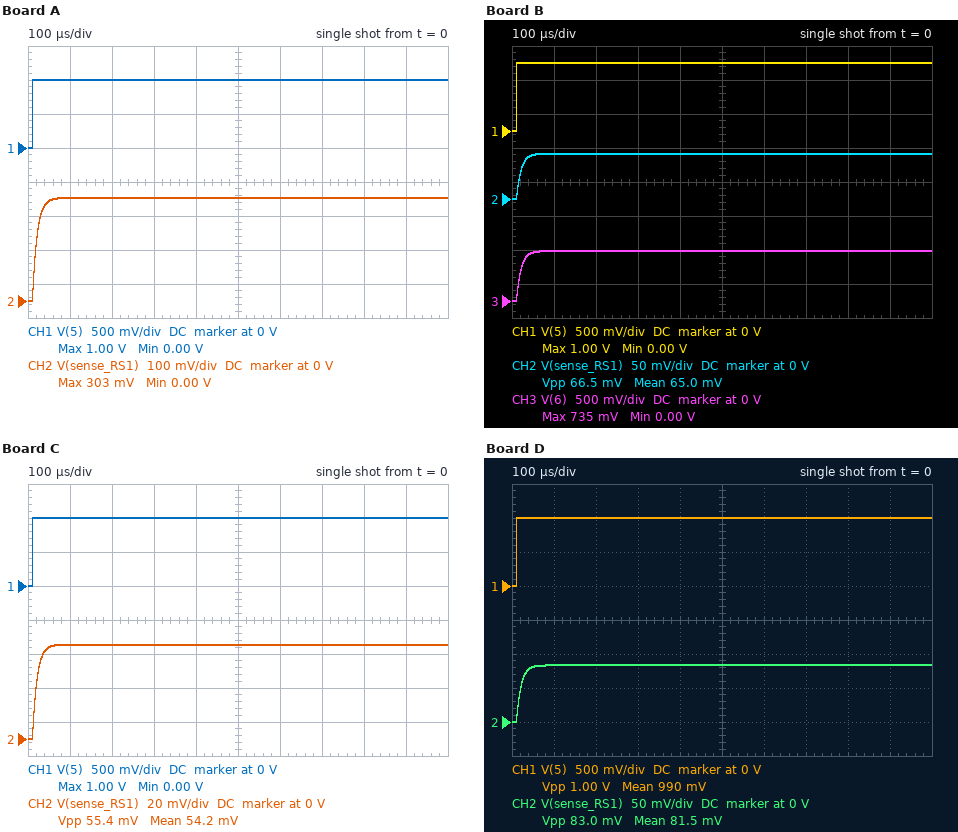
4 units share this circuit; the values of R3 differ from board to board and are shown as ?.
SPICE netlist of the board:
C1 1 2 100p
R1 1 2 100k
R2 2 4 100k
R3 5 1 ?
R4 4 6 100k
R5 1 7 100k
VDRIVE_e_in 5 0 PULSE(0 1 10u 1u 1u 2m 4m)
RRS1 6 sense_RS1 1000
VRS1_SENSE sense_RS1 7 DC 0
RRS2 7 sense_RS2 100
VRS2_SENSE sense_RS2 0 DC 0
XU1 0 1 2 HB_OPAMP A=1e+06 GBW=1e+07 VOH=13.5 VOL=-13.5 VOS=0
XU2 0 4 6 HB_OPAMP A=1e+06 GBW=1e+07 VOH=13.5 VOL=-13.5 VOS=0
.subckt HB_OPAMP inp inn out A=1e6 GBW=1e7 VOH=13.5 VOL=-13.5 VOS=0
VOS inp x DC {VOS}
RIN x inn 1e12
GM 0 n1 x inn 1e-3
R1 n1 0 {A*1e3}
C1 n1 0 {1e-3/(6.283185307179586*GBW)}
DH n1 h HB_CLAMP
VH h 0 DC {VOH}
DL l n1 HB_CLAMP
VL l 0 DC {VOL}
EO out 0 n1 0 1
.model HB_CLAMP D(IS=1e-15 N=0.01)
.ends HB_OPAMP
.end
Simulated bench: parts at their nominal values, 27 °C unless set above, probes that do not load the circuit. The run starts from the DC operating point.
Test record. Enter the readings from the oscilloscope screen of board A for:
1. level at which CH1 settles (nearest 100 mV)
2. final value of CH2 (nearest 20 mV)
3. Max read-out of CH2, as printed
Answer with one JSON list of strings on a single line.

["1.0 V", "300 mV", "303 mV"]
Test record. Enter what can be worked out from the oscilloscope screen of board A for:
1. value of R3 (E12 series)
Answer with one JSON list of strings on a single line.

["33 kΩ"]
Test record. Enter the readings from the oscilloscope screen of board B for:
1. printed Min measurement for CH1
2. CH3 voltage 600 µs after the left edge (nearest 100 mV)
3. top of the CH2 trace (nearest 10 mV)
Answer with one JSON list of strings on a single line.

["0.00 V", "700 mV", "70 mV"]
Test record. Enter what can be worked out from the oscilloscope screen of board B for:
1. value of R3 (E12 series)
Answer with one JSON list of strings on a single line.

["150 kΩ"]
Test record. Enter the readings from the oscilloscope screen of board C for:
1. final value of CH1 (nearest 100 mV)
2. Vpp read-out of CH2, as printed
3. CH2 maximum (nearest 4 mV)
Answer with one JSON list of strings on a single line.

["1.0 V", "55.4 mV", "56 mV"]
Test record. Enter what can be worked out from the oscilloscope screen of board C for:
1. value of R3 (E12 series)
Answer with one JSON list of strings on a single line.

["180 kΩ"]
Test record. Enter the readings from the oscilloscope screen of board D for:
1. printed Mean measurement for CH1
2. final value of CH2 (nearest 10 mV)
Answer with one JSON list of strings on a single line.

["990 mV", "80 mV"]
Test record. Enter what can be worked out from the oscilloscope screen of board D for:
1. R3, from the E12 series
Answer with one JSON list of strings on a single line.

["120 kΩ"]
